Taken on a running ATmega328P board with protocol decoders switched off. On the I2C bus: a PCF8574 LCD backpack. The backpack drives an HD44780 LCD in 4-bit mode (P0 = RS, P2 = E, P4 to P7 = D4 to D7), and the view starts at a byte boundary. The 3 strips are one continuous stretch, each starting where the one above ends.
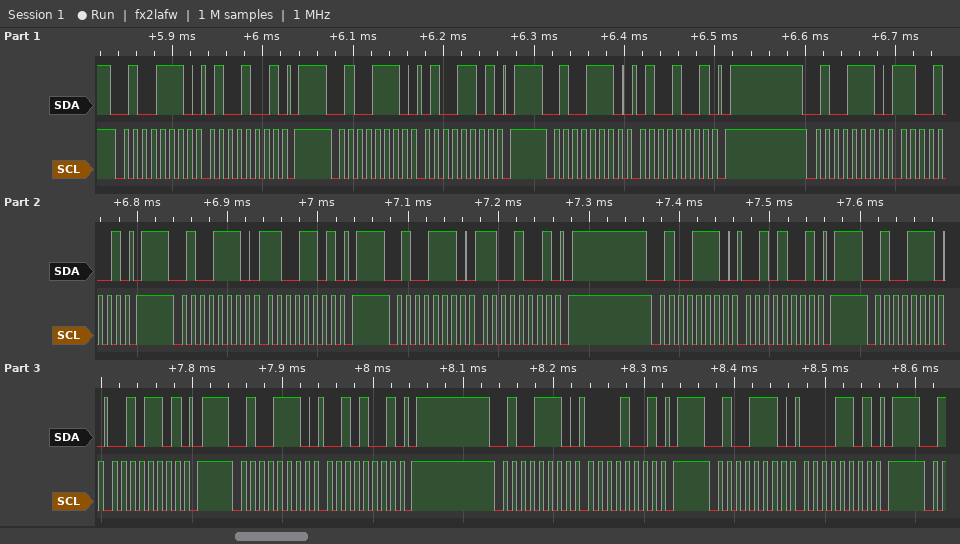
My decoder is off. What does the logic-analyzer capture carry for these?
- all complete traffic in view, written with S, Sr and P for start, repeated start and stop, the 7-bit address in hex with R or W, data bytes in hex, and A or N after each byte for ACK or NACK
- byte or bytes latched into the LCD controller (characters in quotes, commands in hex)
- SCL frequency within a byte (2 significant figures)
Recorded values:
S 27W A 49 A P S 27W A 4D A P S 27W A 49 A P S 27W A C9 A P S 27W A CD A P S 27W A C9 A P S 27W A 29 A P S 27W A 2D A P S 27W A 29 A P S 27W A 09 A P S 27W A 0D A P
'L'
100 kHz
